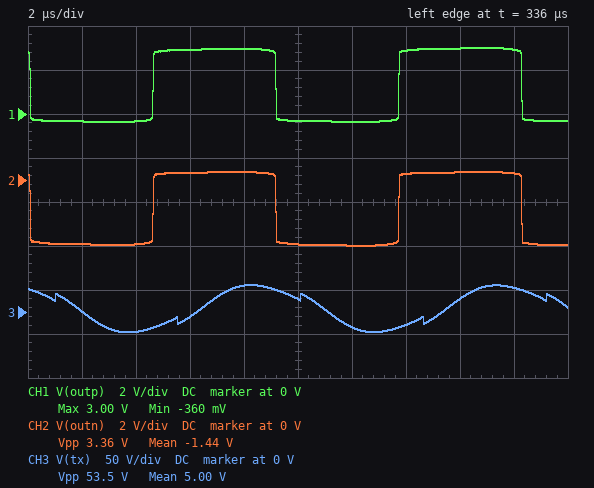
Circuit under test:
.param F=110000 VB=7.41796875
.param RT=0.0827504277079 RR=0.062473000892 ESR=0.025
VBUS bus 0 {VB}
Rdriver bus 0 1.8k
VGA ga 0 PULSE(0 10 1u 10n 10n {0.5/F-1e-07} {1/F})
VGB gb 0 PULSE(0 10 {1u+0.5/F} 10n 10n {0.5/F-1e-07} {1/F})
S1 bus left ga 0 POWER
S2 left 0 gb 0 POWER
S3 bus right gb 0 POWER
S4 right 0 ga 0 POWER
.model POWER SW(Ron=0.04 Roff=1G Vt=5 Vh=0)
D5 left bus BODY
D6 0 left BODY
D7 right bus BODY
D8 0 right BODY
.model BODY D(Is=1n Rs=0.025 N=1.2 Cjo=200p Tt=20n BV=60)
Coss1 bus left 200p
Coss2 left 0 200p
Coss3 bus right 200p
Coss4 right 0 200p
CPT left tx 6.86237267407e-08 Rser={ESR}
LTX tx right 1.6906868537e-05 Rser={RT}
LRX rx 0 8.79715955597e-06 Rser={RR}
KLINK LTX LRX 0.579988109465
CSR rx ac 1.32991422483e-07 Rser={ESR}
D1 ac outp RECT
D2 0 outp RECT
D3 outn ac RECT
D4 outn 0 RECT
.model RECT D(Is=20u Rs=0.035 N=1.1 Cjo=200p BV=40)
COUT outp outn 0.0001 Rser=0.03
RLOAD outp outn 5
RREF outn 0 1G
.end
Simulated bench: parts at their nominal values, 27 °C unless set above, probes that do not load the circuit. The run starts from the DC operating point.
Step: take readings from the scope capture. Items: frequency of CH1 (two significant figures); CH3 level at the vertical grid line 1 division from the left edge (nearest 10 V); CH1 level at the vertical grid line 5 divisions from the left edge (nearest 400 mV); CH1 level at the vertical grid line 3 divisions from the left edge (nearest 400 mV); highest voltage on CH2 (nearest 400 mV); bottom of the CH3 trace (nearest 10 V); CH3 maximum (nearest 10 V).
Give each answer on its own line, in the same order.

110 kHz
0 V
-400 mV
2.8 V
400 mV
-20 V
30 V
